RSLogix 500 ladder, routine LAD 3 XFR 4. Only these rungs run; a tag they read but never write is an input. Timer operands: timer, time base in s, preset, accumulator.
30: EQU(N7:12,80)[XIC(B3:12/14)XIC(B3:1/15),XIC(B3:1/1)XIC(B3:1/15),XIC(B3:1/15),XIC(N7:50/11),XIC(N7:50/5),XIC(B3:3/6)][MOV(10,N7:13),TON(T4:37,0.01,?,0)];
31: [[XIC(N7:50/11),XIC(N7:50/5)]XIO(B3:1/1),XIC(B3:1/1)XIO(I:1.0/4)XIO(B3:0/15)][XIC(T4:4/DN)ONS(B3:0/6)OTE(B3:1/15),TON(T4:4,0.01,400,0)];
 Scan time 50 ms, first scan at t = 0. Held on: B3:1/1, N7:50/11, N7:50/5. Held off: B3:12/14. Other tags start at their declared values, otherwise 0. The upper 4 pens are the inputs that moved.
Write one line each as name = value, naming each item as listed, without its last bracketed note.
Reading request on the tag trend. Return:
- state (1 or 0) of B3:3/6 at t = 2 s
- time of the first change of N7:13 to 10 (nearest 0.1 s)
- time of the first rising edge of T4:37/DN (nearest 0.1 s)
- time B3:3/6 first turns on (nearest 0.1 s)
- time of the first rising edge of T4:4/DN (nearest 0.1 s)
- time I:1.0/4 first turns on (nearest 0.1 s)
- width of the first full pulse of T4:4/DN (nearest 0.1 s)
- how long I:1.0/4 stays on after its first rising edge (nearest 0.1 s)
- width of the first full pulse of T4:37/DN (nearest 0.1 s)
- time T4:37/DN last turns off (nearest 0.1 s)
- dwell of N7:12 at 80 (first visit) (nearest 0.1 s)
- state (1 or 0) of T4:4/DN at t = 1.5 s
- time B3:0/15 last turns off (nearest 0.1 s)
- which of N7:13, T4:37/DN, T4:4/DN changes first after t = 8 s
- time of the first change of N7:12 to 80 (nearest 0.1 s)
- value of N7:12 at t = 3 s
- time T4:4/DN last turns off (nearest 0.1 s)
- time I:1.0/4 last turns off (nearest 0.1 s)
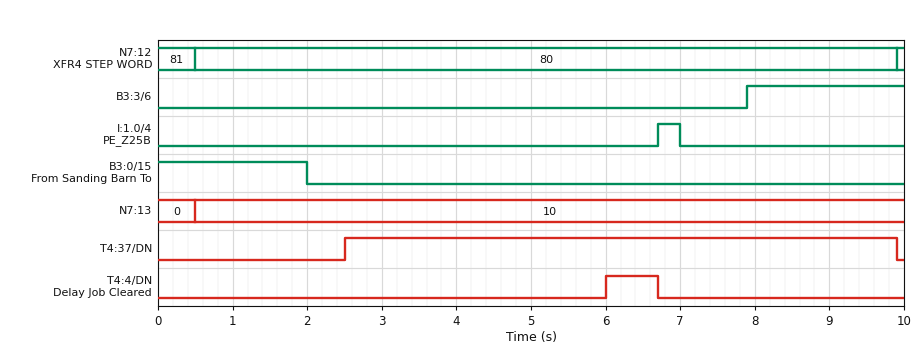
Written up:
state (1 or 0) of B3:3/6 at t = 2 s = 0
time of the first change of N7:13 to 10 = 0.5 s
time of the first rising edge of T4:37/DN = 2.5 s
time B3:3/6 first turns on = 7.9 s
time of the first rising edge of T4:4/DN = 6.0 s
time I:1.0/4 first turns on = 6.7 s
width of the first full pulse of T4:4/DN = 0.7 s
how long I:1.0/4 stays on after its first rising edge = 0.3 s
width of the first full pulse of T4:37/DN = 7.4 s
time T4:37/DN last turns off = 9.9 s
dwell of N7:12 at 80 (first visit) = 9.4 s
state (1 or 0) of T4:4/DN at t = 1.5 s = 0
time B3:0/15 last turns off = 2.0 s
which of N7:13, T4:37/DN, T4:4/DN changes first after t = 8 s = T4:37/DN
time of the first change of N7:12 to 80 = 0.5 s
value of N7:12 at t = 3 s = 80
time T4:4/DN last turns off = 6.7 s
time I:1.0/4 last turns off = 7.0 s
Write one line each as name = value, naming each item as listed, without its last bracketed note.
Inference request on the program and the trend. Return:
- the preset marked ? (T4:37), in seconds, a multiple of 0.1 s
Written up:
the preset marked ? (T4:37), in seconds, a multiple of 0.1 s = 2.0 s
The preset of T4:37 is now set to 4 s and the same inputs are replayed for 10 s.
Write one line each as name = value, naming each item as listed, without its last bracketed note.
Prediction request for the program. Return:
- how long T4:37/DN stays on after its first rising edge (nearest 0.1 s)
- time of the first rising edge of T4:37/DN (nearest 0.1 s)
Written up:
how long T4:37/DN stays on after its first rising edge = 5.4 s
time of the first rising edge of T4:37/DN = 4.5 s
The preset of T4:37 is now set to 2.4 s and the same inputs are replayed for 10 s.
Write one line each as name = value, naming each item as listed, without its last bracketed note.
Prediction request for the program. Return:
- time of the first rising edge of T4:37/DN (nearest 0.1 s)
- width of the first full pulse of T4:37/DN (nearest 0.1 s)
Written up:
time of the first rising edge of T4:37/DN = 2.9 s
width of the first full pulse of T4:37/DN = 7.0 s
